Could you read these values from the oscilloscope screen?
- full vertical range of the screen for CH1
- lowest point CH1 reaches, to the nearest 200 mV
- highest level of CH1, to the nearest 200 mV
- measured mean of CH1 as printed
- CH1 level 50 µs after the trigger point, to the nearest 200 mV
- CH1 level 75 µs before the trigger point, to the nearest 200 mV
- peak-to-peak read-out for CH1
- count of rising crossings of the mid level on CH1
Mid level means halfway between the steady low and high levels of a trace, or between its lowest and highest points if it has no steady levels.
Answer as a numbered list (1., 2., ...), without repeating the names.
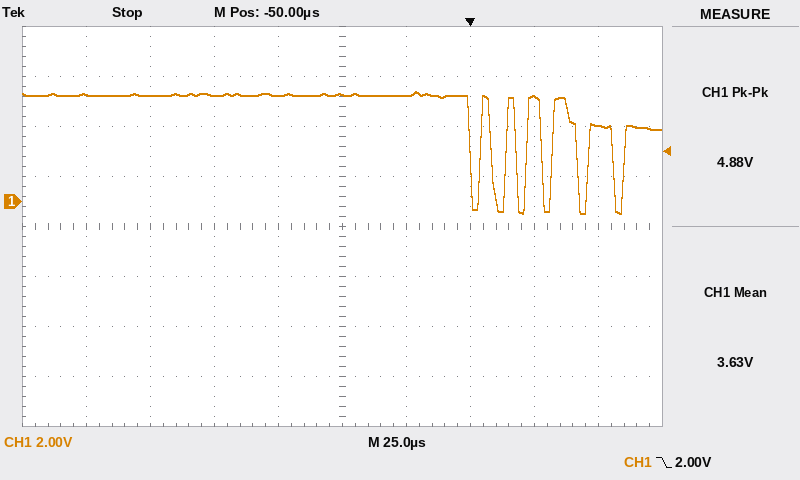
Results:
1. 16 V
2. -400 mV
3. 4.4 V
4. 3.63 V
5. 3.0 V
6. 4.2 V
7. 4.88 V
8. 6
